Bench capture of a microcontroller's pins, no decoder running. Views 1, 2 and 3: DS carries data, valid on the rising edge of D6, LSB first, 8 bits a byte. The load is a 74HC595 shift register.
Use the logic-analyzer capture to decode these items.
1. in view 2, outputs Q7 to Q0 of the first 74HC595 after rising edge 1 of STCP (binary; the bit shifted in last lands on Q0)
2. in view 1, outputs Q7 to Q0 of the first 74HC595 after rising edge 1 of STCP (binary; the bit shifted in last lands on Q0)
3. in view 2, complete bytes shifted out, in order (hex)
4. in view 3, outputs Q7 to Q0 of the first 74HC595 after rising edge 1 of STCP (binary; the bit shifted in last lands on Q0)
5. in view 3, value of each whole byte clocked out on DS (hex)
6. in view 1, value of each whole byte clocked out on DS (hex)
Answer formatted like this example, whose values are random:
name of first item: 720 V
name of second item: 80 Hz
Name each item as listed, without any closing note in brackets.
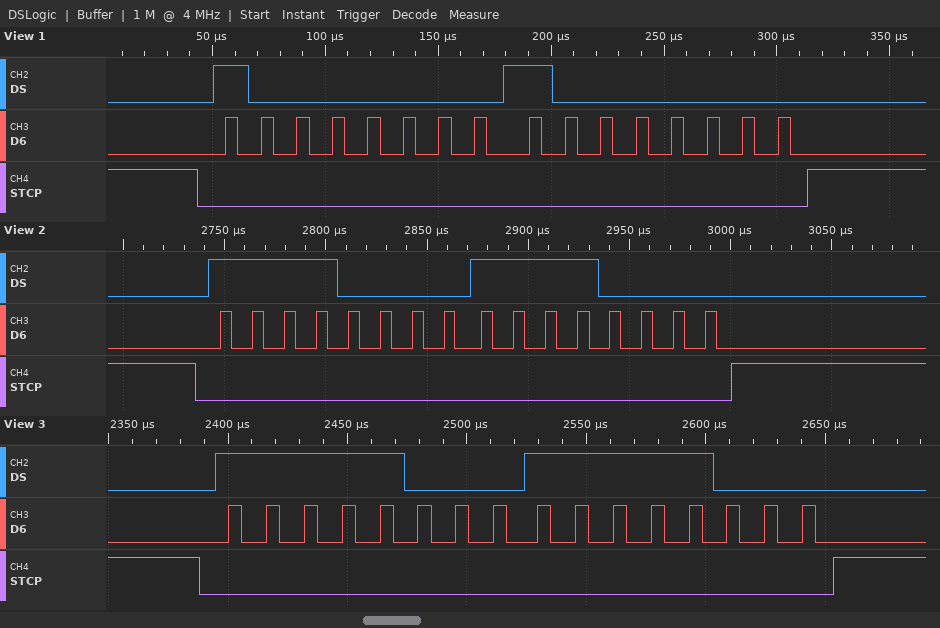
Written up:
in view 2, outputs Q7 to Q0 of the first 74HC595 after rising edge 1 of STCP: 11110000
in view 1, outputs Q7 to Q0 of the first 74HC595 after rising edge 1 of STCP: 10000000
in view 2, complete bytes shifted out, in order: 0F 0F
in view 3, outputs Q7 to Q0 of the first 74HC595 after rising edge 1 of STCP: 11111000
in view 3, value of each whole byte clocked out on DS: 0x1F 0x1F
in view 1, value of each whole byte clocked out on DS: 01 01
